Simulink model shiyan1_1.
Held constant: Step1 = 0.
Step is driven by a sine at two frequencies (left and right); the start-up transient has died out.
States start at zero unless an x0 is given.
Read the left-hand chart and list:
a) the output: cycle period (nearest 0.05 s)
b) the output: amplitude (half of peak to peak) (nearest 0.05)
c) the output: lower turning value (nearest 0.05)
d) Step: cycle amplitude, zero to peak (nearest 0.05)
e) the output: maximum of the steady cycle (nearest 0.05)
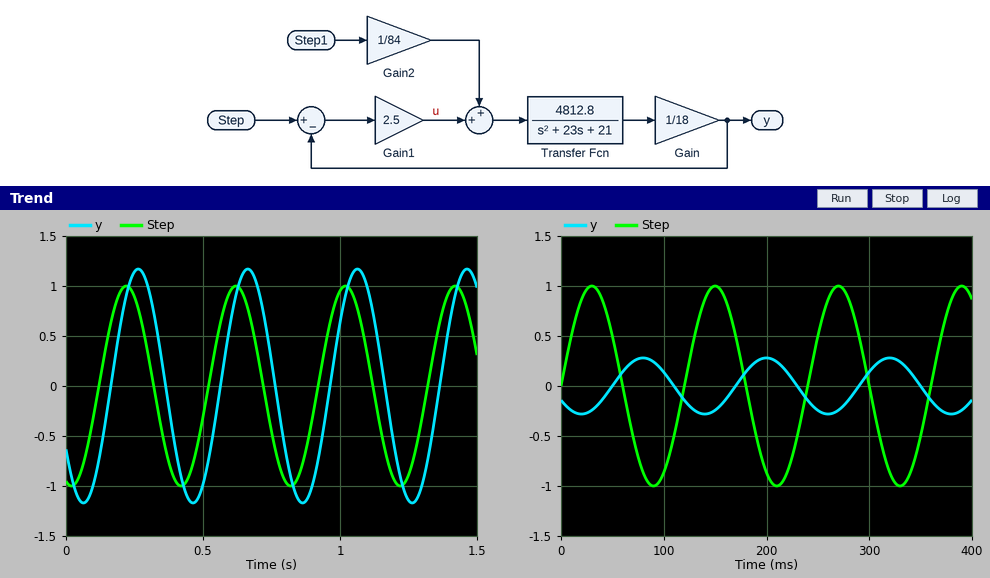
0.40 s
1.15
-1.15
1.00
1.15
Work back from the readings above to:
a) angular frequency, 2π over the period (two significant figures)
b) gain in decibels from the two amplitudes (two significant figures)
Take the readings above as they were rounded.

16 rad/s
1.2 dB
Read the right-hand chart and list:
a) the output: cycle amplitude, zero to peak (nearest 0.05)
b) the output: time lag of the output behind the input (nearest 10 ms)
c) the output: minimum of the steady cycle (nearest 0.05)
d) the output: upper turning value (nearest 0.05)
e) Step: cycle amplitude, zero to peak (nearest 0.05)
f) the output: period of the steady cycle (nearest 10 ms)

0.30
50 ms
-0.30
0.30
1.00
120 ms
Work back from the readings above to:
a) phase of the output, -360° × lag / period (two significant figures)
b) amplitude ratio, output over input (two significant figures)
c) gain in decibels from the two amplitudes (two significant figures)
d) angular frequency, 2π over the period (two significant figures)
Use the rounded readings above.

-150°
0.30
-10 dB
0.052 rad/ms
